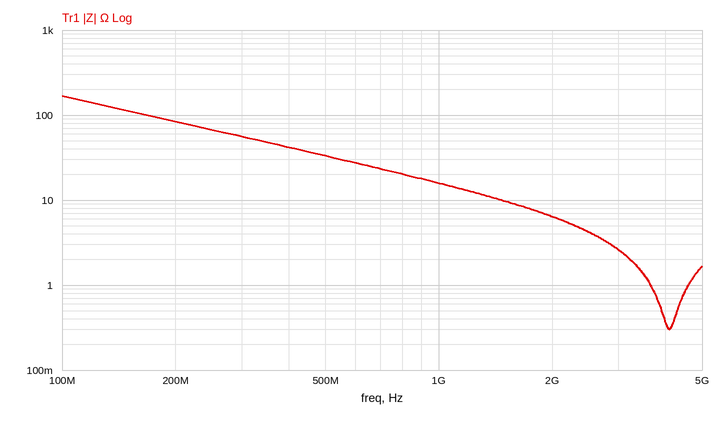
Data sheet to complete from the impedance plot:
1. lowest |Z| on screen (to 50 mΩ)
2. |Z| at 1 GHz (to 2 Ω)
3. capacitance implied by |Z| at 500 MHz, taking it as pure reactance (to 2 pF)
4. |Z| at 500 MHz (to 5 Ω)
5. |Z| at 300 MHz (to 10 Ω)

300 mΩ
16 Ω
10 pF
35 Ω
60 Ω
